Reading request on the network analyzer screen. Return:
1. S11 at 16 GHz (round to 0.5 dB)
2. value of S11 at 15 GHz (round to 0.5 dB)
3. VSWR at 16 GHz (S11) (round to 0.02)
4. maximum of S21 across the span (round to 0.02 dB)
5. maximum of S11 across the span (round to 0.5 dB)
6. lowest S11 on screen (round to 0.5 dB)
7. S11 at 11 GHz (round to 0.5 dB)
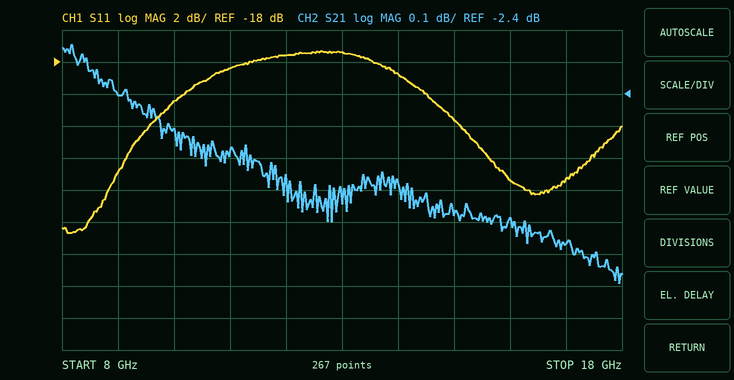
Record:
-25.5 dB
-21.5 dB
1.12
-2.24 dB
-17.5 dB
-28.5 dB
-18.5 dB
